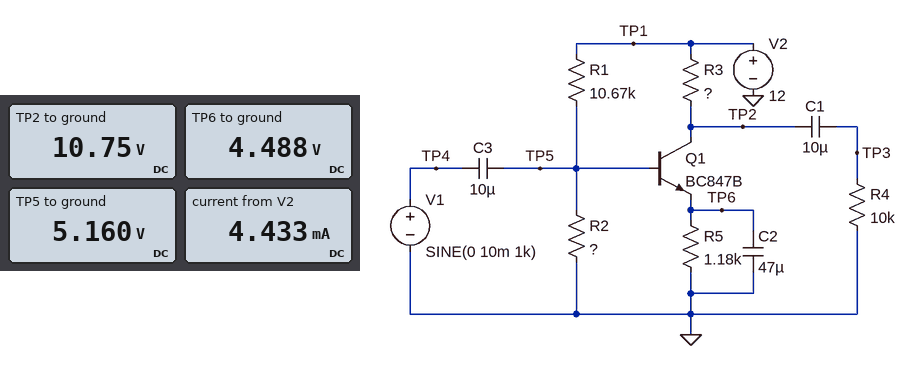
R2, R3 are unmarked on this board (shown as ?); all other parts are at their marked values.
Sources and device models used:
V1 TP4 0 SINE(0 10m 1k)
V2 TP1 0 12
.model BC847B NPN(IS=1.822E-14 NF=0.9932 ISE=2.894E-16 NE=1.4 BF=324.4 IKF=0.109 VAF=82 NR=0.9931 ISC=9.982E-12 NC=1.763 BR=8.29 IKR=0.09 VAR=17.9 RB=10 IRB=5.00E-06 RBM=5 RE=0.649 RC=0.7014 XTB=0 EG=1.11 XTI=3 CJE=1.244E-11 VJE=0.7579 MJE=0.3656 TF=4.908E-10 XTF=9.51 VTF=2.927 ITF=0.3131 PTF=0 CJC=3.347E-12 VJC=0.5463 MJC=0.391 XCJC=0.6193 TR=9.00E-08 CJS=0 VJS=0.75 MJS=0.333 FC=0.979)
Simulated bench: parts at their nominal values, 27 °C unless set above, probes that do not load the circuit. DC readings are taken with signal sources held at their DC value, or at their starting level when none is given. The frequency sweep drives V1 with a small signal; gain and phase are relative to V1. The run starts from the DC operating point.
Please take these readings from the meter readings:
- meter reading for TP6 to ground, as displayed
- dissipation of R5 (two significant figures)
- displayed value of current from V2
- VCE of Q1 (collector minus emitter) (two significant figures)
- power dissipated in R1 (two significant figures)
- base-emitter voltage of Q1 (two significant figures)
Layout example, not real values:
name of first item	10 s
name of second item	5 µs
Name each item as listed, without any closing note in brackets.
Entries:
meter reading for TP6 to ground, as displayed	4.488 V
dissipation of R5	17 mW
displayed value of current from V2	4.433 mA
VCE of Q1 (collector minus emitter)	6.3 V
power dissipated in R1	4.4 mW
base-emitter voltage of Q1	670 mV
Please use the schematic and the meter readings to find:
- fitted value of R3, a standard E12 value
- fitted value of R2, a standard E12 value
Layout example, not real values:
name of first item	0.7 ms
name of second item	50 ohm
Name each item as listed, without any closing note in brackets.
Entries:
fitted value of R3, a standard E12 value	330 Ω
fitted value of R2, a standard E12 value	8.2 kΩ
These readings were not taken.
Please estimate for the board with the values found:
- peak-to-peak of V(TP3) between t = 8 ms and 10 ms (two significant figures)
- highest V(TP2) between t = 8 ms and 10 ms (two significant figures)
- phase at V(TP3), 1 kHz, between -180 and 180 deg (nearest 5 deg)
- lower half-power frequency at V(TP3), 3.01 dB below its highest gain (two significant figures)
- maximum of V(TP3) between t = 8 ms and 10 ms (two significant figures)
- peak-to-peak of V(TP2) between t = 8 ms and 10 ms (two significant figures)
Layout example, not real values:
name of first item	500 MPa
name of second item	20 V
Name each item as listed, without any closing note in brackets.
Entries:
peak-to-peak of V(TP3) between t = 8 ms and 10 ms	740 mV
highest V(TP2) between t = 8 ms and 10 ms	11 V
phase at V(TP3), 1 kHz, between -180 and 180 deg	-155 deg
lower half-power frequency at V(TP3), 3.01 dB below its highest gain	450 Hz
maximum of V(TP3) between t = 8 ms and 10 ms	350 mV
peak-to-peak of V(TP2) between t = 8 ms and 10 ms	740 mV
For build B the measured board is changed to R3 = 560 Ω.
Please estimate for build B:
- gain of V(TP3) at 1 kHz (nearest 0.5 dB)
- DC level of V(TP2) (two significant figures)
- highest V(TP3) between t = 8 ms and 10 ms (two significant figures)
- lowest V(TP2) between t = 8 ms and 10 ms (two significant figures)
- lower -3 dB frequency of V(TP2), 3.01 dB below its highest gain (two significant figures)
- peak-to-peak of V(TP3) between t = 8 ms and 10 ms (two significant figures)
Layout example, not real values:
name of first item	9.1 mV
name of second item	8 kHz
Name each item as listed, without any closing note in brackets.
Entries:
gain of V(TP3) at 1 kHz	36.0 dB
DC level of V(TP2)	9.9 V
highest V(TP3) between t = 8 ms and 10 ms	570 mV
lowest V(TP2) between t = 8 ms and 10 ms	9.2 V
lower -3 dB frequency of V(TP2), 3.01 dB below its highest gain	440 Hz
peak-to-peak of V(TP3) between t = 8 ms and 10 ms	1.2 V
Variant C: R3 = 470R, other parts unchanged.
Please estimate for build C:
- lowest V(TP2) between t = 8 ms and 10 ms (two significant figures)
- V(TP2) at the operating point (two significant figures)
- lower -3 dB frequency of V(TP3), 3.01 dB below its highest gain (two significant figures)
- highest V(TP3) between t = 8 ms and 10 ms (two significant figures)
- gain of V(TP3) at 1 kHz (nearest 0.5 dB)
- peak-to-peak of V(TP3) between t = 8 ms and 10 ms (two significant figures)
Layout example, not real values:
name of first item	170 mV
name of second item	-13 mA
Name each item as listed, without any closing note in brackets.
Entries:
lowest V(TP2) between t = 8 ms and 10 ms	9.7 V
V(TP2) at the operating point	10 V
lower -3 dB frequency of V(TP3), 3.01 dB below its highest gain	440 Hz
highest V(TP3) between t = 8 ms and 10 ms	490 mV
gain of V(TP3) at 1 kHz	34.5 dB
peak-to-peak of V(TP3) between t = 8 ms and 10 ms	1.0 V
